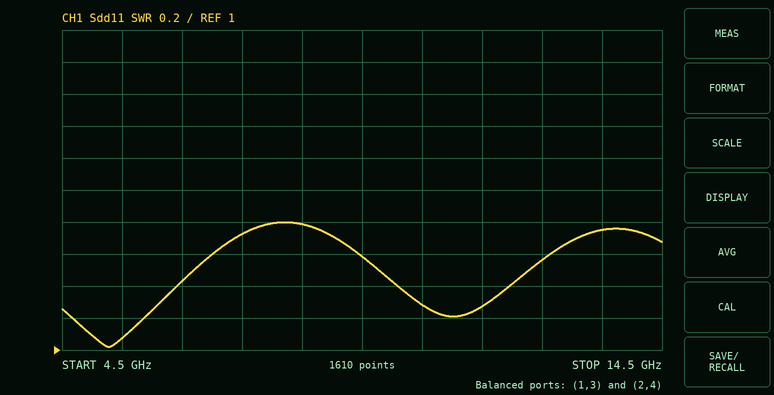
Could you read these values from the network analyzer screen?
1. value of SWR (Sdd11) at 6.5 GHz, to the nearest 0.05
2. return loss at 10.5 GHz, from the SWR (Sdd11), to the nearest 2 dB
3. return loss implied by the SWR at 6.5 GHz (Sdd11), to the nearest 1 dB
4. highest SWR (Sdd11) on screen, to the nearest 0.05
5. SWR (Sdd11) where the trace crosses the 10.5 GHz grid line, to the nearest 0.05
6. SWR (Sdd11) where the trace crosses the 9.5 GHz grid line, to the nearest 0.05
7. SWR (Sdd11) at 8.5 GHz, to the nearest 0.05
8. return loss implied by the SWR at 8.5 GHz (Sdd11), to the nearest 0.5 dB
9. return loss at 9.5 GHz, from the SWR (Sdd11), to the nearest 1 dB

1.45
18 dB
15 dB
1.80
1.30
1.60
1.80
11.0 dB
13 dB
